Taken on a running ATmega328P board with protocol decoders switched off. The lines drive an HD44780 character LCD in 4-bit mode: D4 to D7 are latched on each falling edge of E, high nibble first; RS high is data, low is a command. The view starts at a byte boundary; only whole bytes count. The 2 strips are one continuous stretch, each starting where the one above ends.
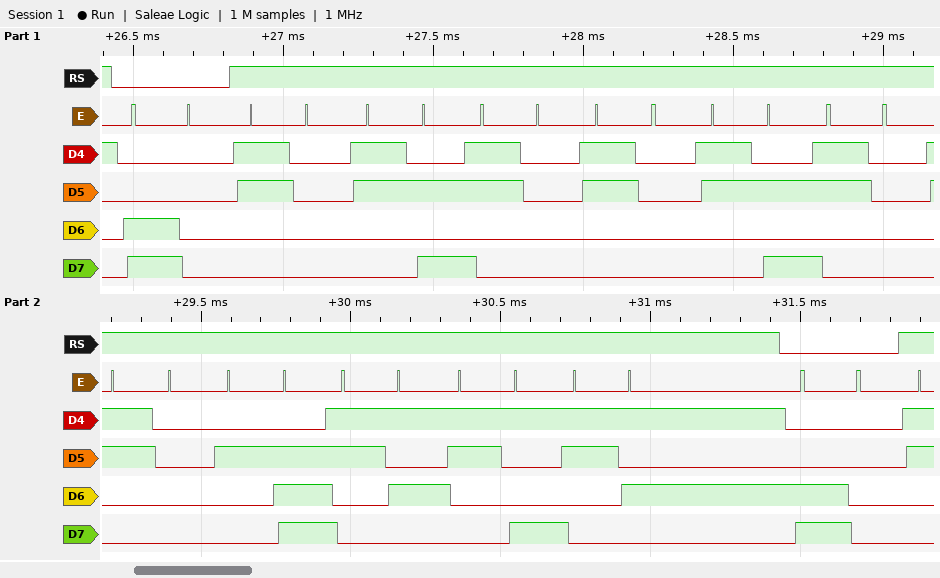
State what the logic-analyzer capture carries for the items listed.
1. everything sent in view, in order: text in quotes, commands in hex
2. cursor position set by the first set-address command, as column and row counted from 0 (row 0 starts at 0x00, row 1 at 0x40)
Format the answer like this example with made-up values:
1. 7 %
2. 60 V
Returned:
1. 0xC0 "0:00:00.595" 0xC0
2. column 0, row 1
